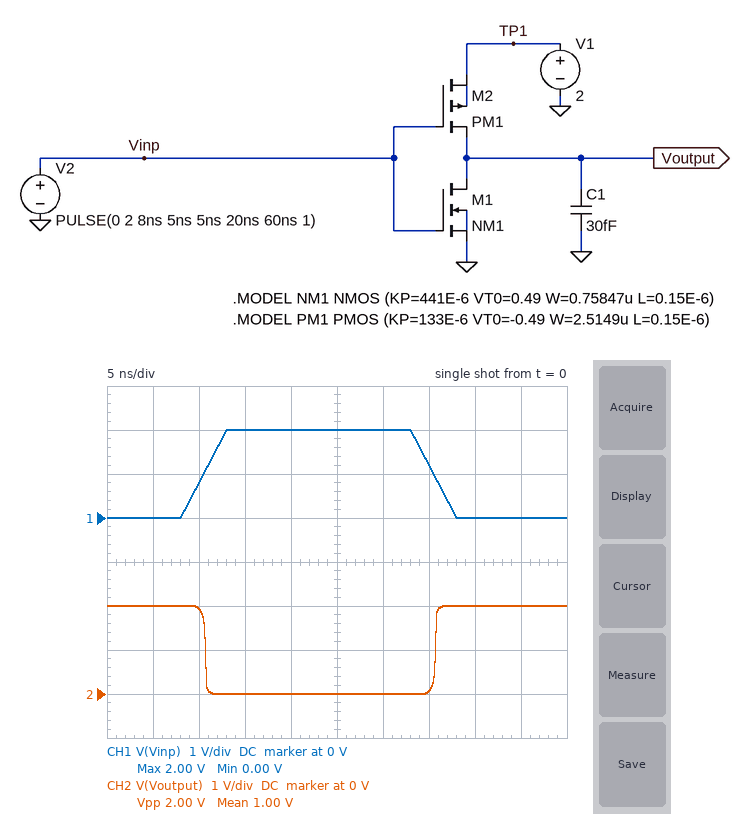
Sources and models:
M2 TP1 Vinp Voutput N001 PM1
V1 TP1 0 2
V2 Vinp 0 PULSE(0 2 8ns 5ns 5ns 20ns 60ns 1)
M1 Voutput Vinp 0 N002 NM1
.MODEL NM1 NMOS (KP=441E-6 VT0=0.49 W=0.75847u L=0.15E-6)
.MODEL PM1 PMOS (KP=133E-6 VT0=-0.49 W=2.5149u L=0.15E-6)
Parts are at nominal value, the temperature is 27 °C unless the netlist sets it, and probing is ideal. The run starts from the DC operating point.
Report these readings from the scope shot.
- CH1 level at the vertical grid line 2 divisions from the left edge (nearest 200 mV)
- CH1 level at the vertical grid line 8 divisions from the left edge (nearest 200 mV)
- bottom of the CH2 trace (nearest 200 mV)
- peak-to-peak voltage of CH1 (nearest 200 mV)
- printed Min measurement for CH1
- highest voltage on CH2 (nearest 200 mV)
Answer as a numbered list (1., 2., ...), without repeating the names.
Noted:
1. 800 mV
2. 0 V
3. 0 V
4. 2.0 V
5. 0.00 V
6. 2.0 V
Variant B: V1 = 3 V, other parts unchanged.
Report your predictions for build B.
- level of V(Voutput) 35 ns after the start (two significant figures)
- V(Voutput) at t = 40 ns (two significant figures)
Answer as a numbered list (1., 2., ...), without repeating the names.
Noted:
1. 2.8 V
2. 3.0 V
